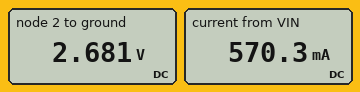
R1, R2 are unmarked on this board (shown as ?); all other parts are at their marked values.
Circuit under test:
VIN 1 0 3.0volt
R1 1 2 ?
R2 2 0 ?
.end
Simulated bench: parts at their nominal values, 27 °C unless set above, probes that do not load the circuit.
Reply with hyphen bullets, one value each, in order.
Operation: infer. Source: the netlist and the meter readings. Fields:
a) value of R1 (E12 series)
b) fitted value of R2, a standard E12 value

- 0.56 Ω
- 4.7 Ω
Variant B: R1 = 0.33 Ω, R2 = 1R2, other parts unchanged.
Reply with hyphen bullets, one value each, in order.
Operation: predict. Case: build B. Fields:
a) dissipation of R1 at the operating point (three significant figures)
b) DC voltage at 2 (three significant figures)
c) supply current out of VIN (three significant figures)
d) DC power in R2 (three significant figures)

- 1.27 W
- 2.35 V
- 1.96 A
- 4.61 W
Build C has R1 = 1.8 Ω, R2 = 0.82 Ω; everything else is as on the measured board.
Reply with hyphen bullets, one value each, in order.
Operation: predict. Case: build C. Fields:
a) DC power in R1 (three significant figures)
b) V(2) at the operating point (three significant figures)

- 2.36 W
- 939 mV
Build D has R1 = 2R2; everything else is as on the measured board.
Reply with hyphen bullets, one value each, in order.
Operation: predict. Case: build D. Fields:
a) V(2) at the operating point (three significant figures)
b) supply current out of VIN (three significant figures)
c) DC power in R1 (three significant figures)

- 2.04 V
- 435 mA
- 416 mW
